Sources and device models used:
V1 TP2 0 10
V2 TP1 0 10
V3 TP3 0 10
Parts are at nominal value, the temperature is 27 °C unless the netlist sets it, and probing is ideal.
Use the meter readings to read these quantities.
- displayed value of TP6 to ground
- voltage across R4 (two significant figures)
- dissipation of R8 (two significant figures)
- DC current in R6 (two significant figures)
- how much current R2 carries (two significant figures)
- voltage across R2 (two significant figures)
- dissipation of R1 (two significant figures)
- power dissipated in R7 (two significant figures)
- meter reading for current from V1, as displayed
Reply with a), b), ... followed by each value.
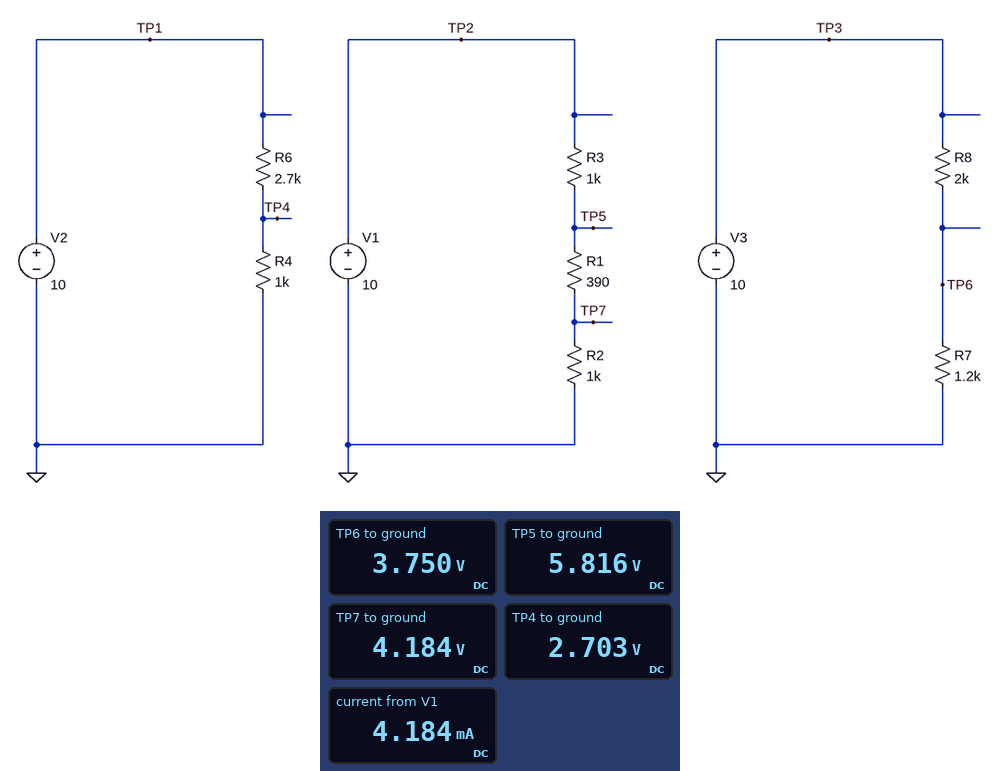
a) 3.750 V
b) 2.7 V
c) 20 mW
d) 2.7 mA
e) 4.2 mA
f) 4.2 V
g) 6.8 mW
h) 12 mW
i) 4.184 mA
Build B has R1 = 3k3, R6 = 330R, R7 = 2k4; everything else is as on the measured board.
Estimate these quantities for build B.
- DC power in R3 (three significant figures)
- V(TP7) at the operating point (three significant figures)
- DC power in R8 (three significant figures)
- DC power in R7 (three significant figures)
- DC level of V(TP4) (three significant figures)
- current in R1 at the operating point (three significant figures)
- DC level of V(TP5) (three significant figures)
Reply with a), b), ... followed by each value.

a) 3.56 mW
b) 1.89 V
c) 10.3 mW
d) 12.4 mW
e) 7.52 V
f) 1.89 mA
g) 8.11 V
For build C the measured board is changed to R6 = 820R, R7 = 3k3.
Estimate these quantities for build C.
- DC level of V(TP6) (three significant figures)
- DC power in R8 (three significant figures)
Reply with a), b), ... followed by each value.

a) 6.23 V
b) 7.12 mW
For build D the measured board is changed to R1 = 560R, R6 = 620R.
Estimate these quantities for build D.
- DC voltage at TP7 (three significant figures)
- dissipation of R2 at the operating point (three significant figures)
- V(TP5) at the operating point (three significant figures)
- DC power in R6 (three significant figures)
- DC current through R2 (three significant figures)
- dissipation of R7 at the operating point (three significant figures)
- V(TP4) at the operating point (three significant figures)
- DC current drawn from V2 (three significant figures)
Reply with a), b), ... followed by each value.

a) 3.91 V
b) 15.3 mW
c) 6.09 V
d) 23.6 mW
e) 3.91 mA
f) 11.7 mW
g) 6.17 V
h) 6.17 mA
